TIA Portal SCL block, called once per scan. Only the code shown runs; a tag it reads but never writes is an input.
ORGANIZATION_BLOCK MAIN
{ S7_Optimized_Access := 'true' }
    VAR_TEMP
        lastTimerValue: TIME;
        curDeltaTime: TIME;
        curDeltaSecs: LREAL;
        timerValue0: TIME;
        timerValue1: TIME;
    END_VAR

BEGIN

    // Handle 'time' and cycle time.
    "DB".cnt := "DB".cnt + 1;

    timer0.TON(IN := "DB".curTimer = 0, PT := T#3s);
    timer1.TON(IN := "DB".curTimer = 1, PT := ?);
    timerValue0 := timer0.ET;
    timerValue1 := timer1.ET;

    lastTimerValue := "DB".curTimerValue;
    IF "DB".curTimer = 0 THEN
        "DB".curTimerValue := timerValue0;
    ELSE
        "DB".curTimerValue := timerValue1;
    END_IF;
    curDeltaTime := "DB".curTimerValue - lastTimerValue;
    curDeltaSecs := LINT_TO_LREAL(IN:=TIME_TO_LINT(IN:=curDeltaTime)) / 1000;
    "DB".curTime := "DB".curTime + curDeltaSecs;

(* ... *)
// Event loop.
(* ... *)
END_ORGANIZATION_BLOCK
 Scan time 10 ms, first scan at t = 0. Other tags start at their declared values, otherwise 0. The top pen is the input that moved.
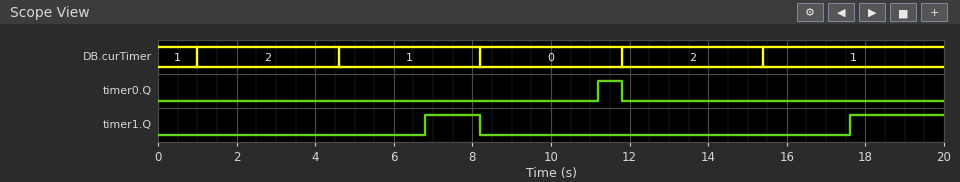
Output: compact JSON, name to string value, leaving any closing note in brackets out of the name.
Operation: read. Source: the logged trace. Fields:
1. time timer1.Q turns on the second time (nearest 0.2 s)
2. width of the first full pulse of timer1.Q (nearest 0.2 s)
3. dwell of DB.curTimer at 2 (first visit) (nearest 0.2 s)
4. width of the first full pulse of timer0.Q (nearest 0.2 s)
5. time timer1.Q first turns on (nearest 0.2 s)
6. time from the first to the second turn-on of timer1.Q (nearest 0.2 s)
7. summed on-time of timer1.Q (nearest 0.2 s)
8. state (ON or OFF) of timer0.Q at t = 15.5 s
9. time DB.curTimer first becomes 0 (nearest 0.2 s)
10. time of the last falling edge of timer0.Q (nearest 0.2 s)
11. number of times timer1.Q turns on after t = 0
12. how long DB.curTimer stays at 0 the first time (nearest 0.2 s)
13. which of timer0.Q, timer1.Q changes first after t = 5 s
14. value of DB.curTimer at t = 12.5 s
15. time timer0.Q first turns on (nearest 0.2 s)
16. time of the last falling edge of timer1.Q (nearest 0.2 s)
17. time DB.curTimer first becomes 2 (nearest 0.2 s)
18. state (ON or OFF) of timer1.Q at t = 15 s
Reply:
{"time timer1.Q turns on the second time": "17.6 s", "width of the first full pulse of timer1.Q": "1.4 s", "dwell of DB.curTimer at 2 (first visit)": "3.6 s", "width of the first full pulse of timer0.Q": "0.6 s", "time timer1.Q first turns on": "6.8 s", "time from the first to the second turn-on of timer1.Q": "10.8 s", "summed on-time of timer1.Q": "3.8 s", "state (ON or OFF) of timer0.Q at t = 15.5 s": "OFF", "time DB.curTimer first becomes 0": "8.2 s", "time of the last falling edge of timer0.Q": "11.8 s", "number of times timer1.Q turns on after t = 0": "2", "how long DB.curTimer stays at 0 the first time": "3.6 s", "which of timer0.Q, timer1.Q changes first after t = 5 s": "timer1.Q", "value of DB.curTimer at t = 12.5 s": "2", "time timer0.Q first turns on": "11.2 s", "time of the last falling edge of timer1.Q": "8.2 s", "time DB.curTimer first becomes 2": "1.0 s", "state (ON or OFF) of timer1.Q at t = 15 s": "OFF"}
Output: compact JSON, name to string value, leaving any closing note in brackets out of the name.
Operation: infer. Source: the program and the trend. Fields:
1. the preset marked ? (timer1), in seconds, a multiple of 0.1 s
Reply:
{"the preset marked ? (timer1), in seconds, a multiple of 0.1 s": "2.2 s"}
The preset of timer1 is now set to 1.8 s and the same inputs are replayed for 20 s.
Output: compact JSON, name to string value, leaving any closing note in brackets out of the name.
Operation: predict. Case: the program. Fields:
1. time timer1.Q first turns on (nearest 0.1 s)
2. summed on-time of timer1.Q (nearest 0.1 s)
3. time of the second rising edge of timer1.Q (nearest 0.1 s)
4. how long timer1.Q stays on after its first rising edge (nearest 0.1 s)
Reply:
{"time timer1.Q first turns on": "6.4 s", "summed on-time of timer1.Q": "4.6 s", "time of the second rising edge of timer1.Q": "17.2 s", "how long timer1.Q stays on after its first rising edge": "1.8 s"}
